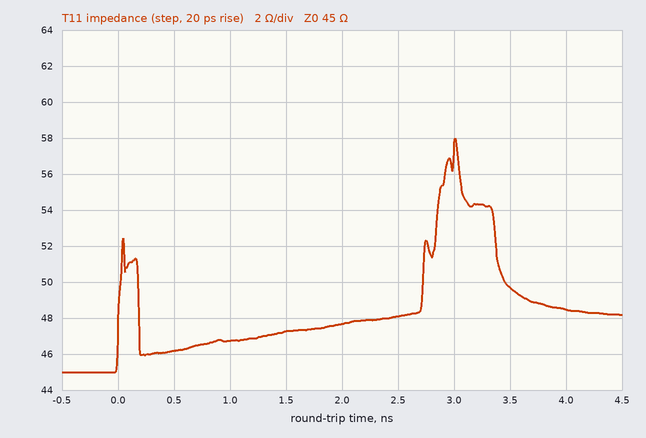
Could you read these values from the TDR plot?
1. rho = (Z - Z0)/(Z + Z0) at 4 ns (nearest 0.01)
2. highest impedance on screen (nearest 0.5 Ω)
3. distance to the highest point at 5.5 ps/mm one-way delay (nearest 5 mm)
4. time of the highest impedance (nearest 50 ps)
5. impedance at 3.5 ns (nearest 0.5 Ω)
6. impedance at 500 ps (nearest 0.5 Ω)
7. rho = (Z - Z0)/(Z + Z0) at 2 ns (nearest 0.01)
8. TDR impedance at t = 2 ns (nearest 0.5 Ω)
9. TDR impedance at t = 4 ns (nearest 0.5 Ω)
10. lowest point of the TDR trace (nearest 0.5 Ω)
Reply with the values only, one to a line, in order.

+0.04
58.0 Ω
275 mm
3.00 ns
49.5 Ω
46.0 Ω
+0.03
47.5 Ω
48.5 Ω
45.0 Ω
